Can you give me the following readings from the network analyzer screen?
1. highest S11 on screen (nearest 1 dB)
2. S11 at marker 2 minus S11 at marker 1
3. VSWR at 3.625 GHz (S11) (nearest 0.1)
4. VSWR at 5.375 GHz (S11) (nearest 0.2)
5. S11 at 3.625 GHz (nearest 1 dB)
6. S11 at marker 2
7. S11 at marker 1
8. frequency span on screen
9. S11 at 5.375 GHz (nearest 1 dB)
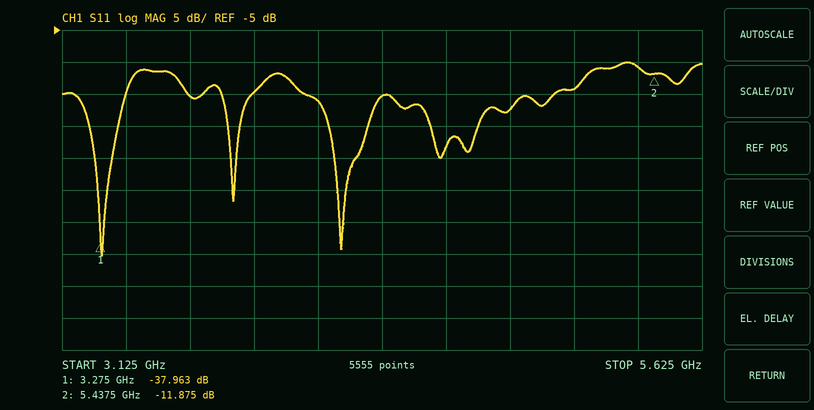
-10 dB
26.088 dB
1.4
1.8
-15 dB
-11.875 dB
-37.963 dB
2.5 GHz
-11 dB
